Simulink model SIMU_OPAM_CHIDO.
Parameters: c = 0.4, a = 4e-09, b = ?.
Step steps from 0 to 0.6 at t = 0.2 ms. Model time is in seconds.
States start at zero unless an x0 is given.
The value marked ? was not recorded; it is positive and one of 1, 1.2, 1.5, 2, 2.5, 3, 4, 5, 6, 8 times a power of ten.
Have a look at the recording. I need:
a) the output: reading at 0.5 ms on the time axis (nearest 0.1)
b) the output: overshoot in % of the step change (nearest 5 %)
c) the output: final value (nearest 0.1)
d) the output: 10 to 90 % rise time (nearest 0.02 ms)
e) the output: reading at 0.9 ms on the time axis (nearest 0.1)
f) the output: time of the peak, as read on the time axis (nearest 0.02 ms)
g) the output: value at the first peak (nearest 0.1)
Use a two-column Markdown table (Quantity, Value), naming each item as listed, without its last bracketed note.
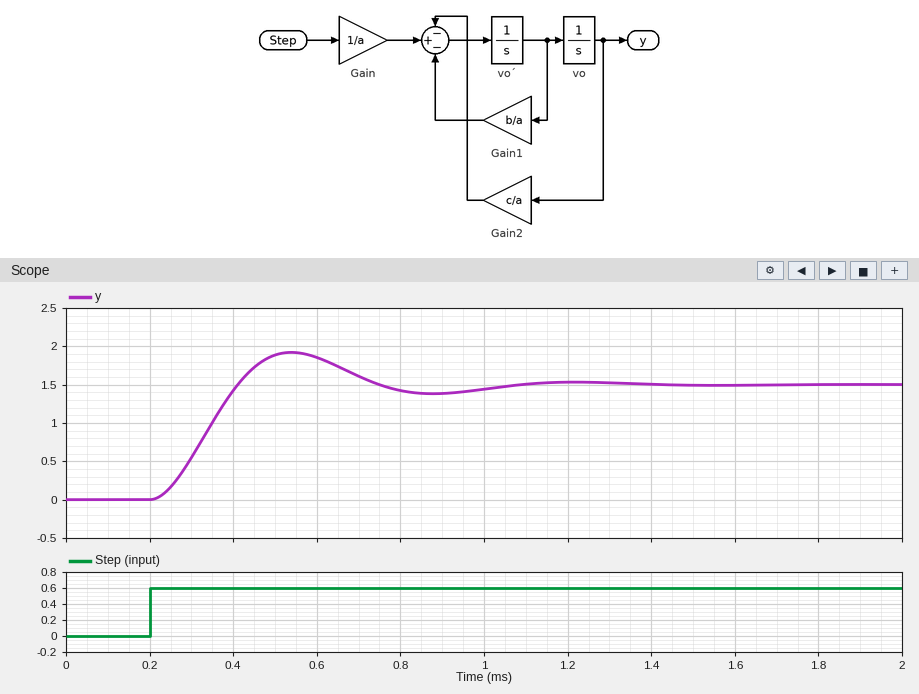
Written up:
| Quantity | Value |
|---|---|
| the output: reading at 0.5 ms on the time axis | 1.9 |
| the output: overshoot in % of the step change | 30 % |
| the output: final value | 1.5 |
| the output: 10 to 90 % rise time | 0.14 ms |
| the output: reading at 0.9 ms on the time axis | 1.4 |
| the output: time of the peak, as read on the time axis | 0.54 ms |
| the output: value at the first peak | 1.9 |
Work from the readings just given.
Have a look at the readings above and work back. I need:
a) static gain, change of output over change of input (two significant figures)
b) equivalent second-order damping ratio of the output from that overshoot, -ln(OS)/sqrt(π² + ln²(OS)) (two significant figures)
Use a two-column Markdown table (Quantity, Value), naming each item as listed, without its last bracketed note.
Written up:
| Quantity | Value |
|---|---|
| static gain, change of output over change of input | 2.5 |
| equivalent second-order damping ratio of the output from that overshoot, -ln(OS)/sqrt(π² + ln²(OS)) | 0.36 |
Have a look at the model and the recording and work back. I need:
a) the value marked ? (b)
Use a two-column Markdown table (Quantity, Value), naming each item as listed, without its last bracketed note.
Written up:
| Quantity | Value |
|---|---|
| the value marked ? | 3e-05 |
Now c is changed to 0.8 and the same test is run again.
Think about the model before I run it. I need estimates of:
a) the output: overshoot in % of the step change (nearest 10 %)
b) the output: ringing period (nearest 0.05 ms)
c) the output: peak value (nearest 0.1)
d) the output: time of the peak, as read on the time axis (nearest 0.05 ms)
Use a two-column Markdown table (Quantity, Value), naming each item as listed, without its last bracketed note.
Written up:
| Quantity | Value |
|---|---|
| the output: overshoot in % of the step change | 40 % |
| the output: ringing period | 0.45 ms |
| the output: peak value | 1.1 |
| the output: time of the peak, as read on the time axis | 0.45 ms |
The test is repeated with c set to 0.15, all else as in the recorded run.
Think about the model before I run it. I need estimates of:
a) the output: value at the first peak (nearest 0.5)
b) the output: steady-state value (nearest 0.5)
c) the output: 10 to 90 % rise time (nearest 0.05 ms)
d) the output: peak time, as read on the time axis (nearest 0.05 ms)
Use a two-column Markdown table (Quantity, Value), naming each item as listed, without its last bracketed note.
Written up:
| Quantity | Value |
|---|---|
| the output: value at the first peak | 4.5 |
| the output: steady-state value | 4.0 |
| the output: 10 to 90 % rise time | 0.30 ms |
| the output: peak time, as read on the time axis | 0.85 ms |
